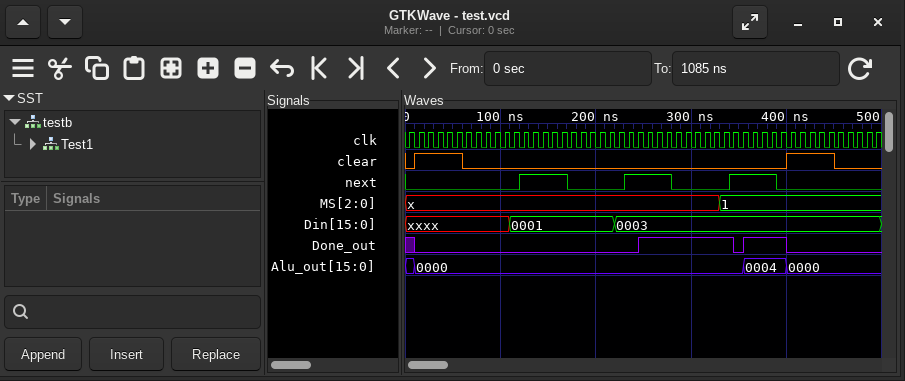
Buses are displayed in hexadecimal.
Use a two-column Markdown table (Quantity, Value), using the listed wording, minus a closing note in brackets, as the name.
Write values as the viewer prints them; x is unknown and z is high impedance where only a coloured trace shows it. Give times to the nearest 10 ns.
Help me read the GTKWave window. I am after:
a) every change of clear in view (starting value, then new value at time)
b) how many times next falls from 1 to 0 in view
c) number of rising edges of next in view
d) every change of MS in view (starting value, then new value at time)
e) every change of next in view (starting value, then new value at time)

| Quantity | Value |
|---|---|
| every change of clear in view | 0, 1 at 10 ns, 0 at 60 ns, 1 at 400 ns, 0 at 450 ns |
| how many times next falls from 1 to 0 in view | 3 |
| number of rising edges of next in view | 3 |
| every change of MS in view | x, 1 at 330 ns |
| every change of next in view | 0, 1 at 120 ns, 0 at 170 ns, 1 at 230 ns, 0 at 280 ns, 1 at 340 ns, 0 at 390 ns |
